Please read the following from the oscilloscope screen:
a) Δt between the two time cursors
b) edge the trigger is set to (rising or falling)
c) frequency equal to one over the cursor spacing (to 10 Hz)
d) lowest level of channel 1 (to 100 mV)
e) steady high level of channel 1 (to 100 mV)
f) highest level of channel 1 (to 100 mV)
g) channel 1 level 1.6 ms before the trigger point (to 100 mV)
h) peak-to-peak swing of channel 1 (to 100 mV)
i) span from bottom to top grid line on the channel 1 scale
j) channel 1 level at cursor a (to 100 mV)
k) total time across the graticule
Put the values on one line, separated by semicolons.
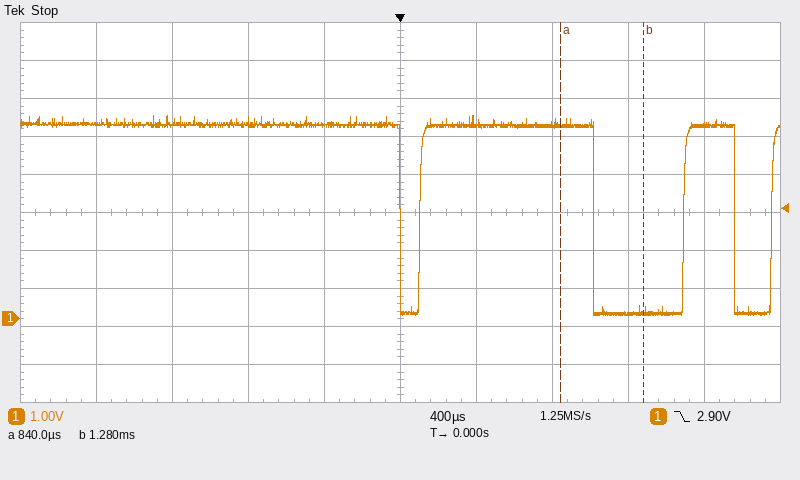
440 µs; falling; 2.27 kHz; 100 mV; 5.1 V; 5.4 V; 5.1 V; 5.3 V; 10 V; 5.1 V; 4 ms
